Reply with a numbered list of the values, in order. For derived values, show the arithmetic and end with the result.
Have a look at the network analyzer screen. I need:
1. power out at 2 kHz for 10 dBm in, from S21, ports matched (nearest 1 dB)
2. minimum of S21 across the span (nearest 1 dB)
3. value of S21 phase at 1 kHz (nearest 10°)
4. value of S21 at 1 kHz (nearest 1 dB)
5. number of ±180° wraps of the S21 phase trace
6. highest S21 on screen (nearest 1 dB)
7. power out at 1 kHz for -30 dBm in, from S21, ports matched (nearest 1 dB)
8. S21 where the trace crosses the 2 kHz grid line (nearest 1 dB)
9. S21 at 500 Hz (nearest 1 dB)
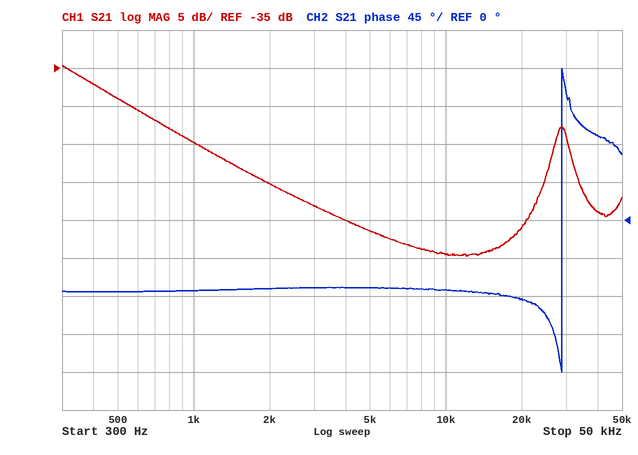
1. 10 dBm + (-50 dB) = -40 dBm
2. -60 dB
3. -80°
4. -45 dB
5. 1
6. -35 dB
7. -30 dBm + (-45 dB) = -75 dBm
8. -50 dB
9. -39 dB
